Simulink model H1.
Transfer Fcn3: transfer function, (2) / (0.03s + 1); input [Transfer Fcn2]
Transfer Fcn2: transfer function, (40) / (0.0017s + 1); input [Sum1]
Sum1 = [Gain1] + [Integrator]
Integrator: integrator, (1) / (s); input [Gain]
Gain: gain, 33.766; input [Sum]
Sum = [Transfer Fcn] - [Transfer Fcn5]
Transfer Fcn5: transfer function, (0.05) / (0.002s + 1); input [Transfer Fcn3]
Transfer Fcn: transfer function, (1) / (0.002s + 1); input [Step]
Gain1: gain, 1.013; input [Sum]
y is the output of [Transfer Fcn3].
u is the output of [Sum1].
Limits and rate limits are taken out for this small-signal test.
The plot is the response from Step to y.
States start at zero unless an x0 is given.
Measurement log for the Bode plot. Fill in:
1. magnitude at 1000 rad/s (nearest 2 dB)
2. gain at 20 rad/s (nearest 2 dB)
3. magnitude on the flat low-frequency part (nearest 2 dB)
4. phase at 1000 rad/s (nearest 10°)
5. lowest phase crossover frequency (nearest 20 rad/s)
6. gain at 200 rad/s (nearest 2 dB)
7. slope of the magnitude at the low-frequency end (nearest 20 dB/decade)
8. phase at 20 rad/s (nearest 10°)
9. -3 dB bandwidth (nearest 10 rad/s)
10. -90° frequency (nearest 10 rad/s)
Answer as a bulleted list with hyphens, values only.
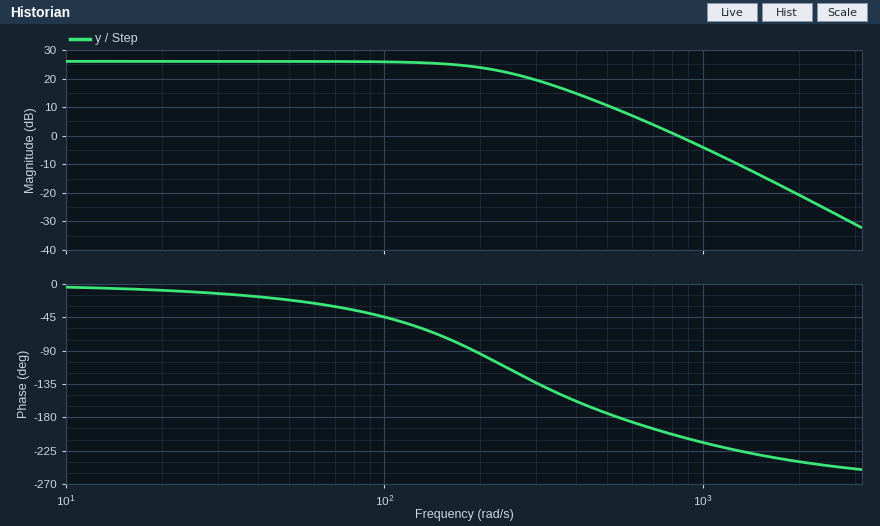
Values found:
- -4 dB
- 26 dB
- 26 dB
- -210°
- 540 rad/s
- 24 dB
- 0 dB/decade
- -10°
- 220 rad/s
- 190 rad/s
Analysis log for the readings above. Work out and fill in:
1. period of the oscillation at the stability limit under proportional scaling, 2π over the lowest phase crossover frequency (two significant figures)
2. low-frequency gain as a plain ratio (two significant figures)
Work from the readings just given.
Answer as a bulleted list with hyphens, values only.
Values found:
- 0.012 s
- 20
